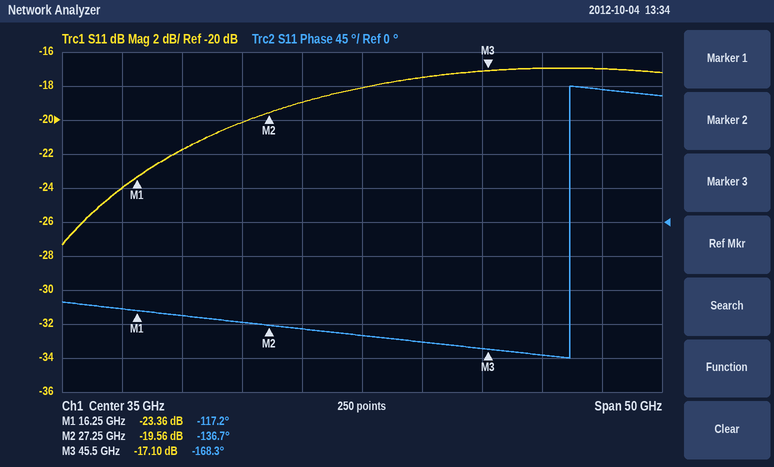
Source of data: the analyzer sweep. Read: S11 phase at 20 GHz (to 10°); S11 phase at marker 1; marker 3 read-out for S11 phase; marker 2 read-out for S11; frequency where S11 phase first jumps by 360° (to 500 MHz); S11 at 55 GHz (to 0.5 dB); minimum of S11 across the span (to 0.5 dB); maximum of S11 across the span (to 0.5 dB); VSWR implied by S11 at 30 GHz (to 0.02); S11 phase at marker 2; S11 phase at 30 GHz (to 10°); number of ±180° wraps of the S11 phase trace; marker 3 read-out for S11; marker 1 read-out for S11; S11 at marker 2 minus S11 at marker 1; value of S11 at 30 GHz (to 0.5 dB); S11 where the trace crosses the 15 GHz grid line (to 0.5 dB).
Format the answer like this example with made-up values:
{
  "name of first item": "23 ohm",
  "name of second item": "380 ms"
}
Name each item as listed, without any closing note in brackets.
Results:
{
  "S11 phase at 20 GHz": "-120°",
  "S11 phase at marker 1": "-117.2°",
  "marker 3 read-out for S11 phase": "-168.3°",
  "marker 2 read-out for S11": "-19.56 dB",
  "frequency where S11 phase first jumps by 360°": "52.5 GHz",
  "S11 at 55 GHz": "-17.0 dB",
  "minimum of S11 across the span": "-27.5 dB",
  "maximum of S11 across the span": "-17.0 dB",
  "VSWR implied by S11 at 30 GHz": "1.26",
  "S11 phase at marker 2": "-136.7°",
  "S11 phase at 30 GHz": "-140°",
  "number of ±180° wraps of the S11 phase trace": "1",
  "marker 3 read-out for S11": "-17.10 dB",
  "marker 1 read-out for S11": "-23.36 dB",
  "S11 at marker 2 minus S11 at marker 1": "3.80 dB",
  "value of S11 at 30 GHz": "-19.0 dB",
  "S11 where the trace crosses the 15 GHz grid line": "-24.0 dB"
}
